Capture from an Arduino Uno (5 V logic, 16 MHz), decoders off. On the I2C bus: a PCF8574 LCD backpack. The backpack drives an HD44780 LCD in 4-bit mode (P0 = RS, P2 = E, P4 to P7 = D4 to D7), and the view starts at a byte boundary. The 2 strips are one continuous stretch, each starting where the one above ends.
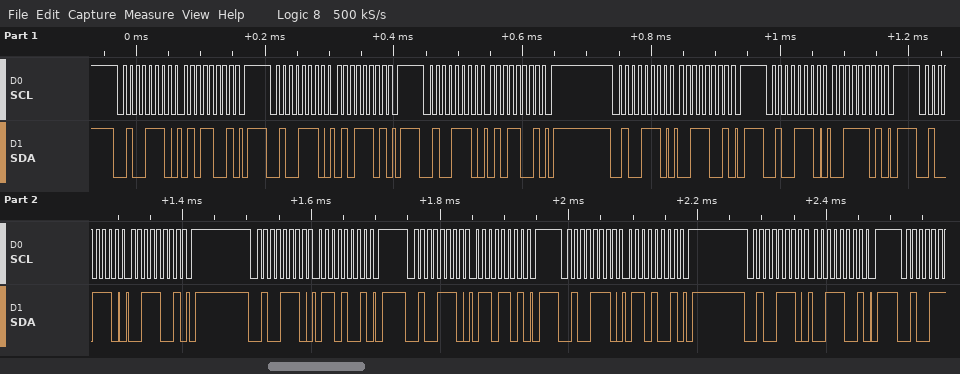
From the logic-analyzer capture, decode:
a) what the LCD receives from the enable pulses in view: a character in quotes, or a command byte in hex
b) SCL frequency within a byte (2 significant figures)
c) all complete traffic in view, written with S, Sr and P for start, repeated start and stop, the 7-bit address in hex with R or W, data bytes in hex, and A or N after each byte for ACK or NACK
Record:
'S'
100 kHz
S 27W A 59 A P S 27W A 5D A P S 27W A 59 A P S 27W A 39 A P S 27W A 3D A P S 27W A 39 A P S 27W A 69 A P S 27W A 6D A P S 27W A 69 A P S 27W A 39 A P
